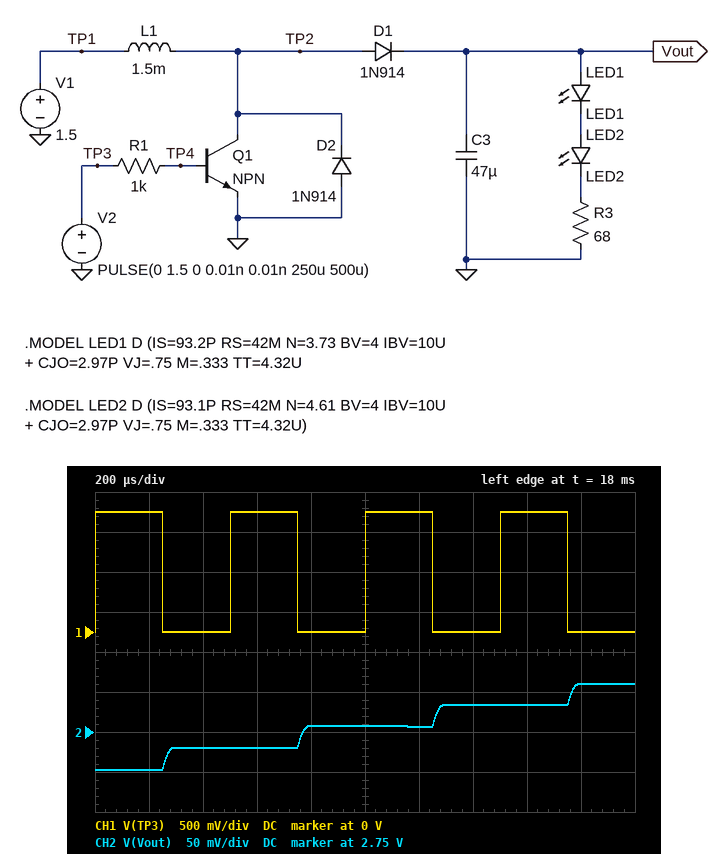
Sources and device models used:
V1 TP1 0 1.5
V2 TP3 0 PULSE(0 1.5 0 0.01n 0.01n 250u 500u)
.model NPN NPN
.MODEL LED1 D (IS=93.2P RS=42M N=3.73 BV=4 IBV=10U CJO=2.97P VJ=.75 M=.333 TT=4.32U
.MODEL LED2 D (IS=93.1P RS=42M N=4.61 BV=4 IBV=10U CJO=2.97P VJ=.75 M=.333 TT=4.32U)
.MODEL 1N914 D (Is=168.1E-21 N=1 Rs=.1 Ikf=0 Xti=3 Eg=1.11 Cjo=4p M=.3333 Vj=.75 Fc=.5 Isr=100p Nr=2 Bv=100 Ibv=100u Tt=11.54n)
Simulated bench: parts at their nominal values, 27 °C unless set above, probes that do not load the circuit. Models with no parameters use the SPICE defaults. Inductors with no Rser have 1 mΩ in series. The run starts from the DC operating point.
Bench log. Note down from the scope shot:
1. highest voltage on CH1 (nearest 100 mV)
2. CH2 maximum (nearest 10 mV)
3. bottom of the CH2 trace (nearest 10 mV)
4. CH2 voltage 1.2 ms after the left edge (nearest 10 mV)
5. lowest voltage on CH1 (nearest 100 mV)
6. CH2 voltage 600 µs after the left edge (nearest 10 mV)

1.5 V
2.81 V
2.70 V
2.76 V
0 V
2.73 V
